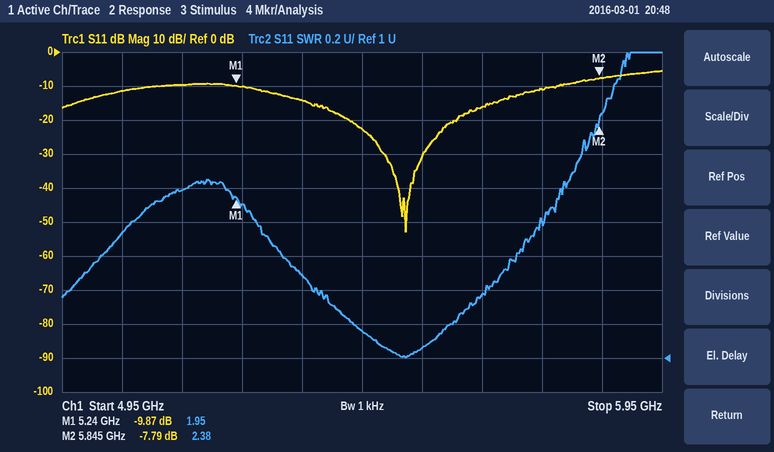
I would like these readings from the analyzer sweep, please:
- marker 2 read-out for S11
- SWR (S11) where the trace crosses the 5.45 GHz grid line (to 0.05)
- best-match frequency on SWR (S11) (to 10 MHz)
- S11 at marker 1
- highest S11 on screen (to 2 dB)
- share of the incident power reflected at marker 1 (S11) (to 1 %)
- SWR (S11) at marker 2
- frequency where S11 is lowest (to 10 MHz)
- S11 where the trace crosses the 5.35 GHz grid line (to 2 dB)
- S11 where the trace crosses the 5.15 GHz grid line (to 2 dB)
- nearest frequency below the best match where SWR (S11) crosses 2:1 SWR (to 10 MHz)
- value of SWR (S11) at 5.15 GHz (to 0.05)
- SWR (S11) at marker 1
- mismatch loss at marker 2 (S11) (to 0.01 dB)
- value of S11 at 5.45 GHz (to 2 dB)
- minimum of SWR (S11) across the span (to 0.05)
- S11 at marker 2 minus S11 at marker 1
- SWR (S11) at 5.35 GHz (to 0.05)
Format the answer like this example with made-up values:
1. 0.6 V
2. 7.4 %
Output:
1. -7.79 dB
2. 1.15
3. 5.52 GHz
4. -9.87 dB
5. -6 dB
6. 10 %
7. 2.38
8. 5.52 GHz
9. -14 dB
10. -10 dB
11. 5.22 GHz
12. 2.00
13. 1.95
14. 0.79 dB
15. -22 dB
16. 1.00
17. 2.08 dB
18. 1.50
